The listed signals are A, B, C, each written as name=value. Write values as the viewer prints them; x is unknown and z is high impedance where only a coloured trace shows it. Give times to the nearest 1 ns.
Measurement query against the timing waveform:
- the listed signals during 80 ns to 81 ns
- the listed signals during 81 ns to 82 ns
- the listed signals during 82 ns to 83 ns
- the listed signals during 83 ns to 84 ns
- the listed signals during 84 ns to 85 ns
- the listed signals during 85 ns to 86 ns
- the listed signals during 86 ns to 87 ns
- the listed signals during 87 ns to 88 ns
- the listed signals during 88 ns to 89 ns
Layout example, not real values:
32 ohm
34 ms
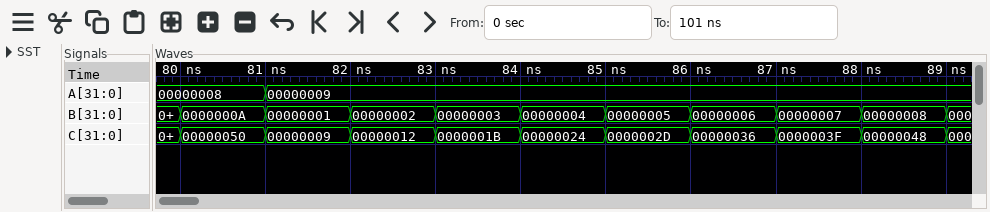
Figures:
A=00000008, B=0000000A, C=00000050
A=00000009, B=00000001, C=00000009
A=00000009, B=00000002, C=00000012
A=00000009, B=00000003, C=0000001B
A=00000009, B=00000004, C=00000024
A=00000009, B=00000005, C=0000002D
A=00000009, B=00000006, C=00000036
A=00000009, B=00000007, C=0000003F
A=00000009, B=00000008, C=00000048
